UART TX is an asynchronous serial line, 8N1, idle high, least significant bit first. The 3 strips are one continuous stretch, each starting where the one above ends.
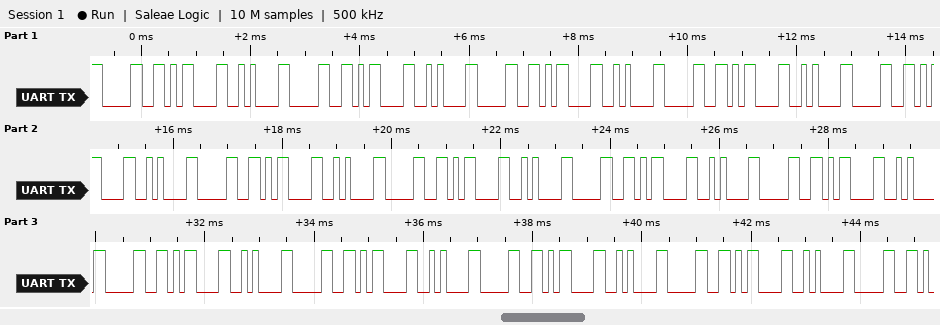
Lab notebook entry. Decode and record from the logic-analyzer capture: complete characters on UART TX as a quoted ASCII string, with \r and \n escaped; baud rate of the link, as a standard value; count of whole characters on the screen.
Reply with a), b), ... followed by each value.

a) "0\r\n0\r\n0\r\n0\r\n0\r\n0\r\n0\r\n0\r\n0\r\n0\r\n0\r\n0\r\n0\r\n0"
b) 9600 baud
c) 40
